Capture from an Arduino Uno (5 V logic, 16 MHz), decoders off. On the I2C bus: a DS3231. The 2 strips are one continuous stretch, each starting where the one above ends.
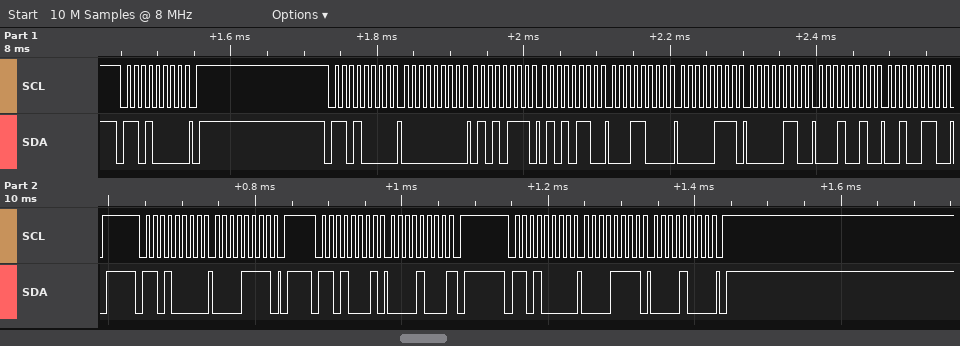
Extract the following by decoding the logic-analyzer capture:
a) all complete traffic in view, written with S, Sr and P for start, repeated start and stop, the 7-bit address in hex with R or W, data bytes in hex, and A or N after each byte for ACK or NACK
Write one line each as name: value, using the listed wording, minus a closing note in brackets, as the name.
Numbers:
all complete traffic in view, written with S, Sr and P for start, repeated start and stop, the 7-bit address in hex with R or W, data bytes in hex, and A or N after each byte for ACK or NACK: S 68W A P S 68W A 00 A 57 A 56 A 18 A 07 A 06 A 12 A 26 A P S 68W A 0F A P S 68R A 08 N P S 68W A 0F A 08 A P
